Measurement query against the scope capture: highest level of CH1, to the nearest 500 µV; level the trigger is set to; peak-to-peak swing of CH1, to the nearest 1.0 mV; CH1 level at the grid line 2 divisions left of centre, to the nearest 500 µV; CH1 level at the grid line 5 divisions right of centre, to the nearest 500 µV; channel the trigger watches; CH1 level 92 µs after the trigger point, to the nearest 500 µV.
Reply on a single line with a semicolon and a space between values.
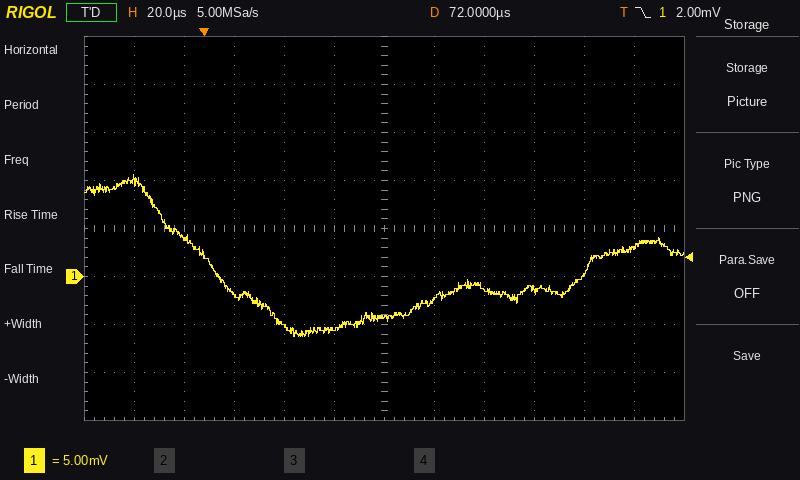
10.5 mV; 2.00 mV; 17.0 mV; -5.0 mV; 3.0 mV; CH1; -2.5 mV
